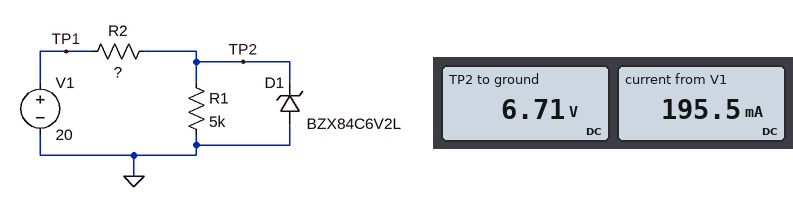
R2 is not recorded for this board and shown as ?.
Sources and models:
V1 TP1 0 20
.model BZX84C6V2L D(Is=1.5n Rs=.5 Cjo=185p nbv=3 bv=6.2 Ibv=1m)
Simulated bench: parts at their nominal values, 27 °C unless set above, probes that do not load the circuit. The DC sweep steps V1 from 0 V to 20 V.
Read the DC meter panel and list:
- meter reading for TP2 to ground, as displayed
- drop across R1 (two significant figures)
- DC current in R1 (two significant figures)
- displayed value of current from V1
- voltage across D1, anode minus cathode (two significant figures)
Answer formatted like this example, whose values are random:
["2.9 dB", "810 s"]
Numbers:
["6.71 V", "6.7 V", "1.3 mA", "195.5 mA", "-6.7 V"]
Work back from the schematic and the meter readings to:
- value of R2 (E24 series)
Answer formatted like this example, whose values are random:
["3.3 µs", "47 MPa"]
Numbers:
["68 Ω"]
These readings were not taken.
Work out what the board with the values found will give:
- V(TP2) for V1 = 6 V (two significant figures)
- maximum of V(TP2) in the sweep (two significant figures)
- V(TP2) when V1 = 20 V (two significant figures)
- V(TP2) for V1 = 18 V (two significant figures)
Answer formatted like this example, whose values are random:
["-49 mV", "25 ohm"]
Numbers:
["5.9 V", "6.7 V", "6.7 V", "6.7 V"]
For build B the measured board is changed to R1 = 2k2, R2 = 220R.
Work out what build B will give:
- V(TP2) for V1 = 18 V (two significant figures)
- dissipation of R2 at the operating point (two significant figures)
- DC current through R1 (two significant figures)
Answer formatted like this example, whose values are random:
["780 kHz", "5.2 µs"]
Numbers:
["6.5 V", "820 mW", "3.0 mA"]
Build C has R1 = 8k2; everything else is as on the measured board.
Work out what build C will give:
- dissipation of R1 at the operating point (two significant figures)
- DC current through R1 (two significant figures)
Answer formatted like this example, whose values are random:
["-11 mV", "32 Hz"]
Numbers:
["5.5 mW", "820 µA"]
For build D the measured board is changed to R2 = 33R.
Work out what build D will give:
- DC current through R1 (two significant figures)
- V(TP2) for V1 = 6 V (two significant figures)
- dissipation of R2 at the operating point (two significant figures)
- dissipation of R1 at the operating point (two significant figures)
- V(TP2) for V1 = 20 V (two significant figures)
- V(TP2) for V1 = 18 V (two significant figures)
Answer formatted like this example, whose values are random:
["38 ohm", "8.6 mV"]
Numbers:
["1.4 mA", "6.0 V", "5.2 W", "9.4 mW", "6.9 V", "6.8 V"]
